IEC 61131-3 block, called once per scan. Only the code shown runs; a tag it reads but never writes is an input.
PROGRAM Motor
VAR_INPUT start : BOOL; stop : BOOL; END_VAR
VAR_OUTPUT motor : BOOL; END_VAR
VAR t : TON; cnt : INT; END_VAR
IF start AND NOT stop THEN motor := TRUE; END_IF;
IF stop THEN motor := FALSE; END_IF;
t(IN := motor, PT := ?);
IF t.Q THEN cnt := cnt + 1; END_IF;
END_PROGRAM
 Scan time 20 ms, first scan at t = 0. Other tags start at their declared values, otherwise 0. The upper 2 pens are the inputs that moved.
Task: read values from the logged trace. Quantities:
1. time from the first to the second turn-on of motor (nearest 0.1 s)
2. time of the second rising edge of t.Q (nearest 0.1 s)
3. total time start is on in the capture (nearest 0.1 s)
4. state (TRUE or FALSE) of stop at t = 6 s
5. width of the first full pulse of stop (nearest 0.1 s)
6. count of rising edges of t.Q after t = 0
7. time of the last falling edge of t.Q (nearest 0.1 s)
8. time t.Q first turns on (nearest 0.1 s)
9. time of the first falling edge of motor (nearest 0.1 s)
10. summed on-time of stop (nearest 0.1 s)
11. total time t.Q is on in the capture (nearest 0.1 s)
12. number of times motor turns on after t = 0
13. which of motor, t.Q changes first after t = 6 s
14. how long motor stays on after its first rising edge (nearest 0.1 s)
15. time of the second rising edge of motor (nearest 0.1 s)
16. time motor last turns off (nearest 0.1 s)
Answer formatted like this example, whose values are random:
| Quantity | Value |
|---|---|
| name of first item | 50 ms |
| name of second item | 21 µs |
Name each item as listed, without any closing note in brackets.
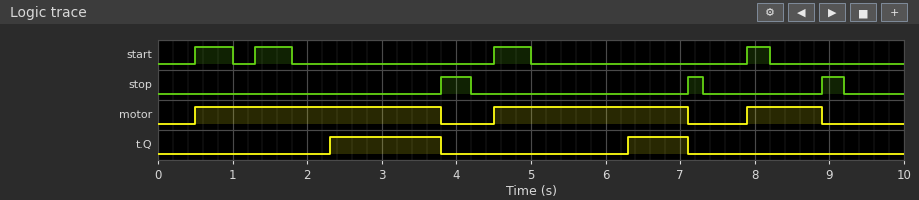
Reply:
| Quantity | Value |
|---|---|
| time from the first to the second turn-on of motor | 4.0 s |
| time of the second rising edge of t.Q | 6.3 s |
| total time start is on in the capture | 1.8 s |
| state (TRUE or FALSE) of stop at t = 6 s | FALSE |
| width of the first full pulse of stop | 0.4 s |
| count of rising edges of t.Q after t = 0 | 2 |
| time of the last falling edge of t.Q | 7.1 s |
| time t.Q first turns on | 2.3 s |
| time of the first falling edge of motor | 3.8 s |
| summed on-time of stop | 0.9 s |
| total time t.Q is on in the capture | 2.3 s |
| number of times motor turns on after t = 0 | 3 |
| which of motor, t.Q changes first after t = 6 s | t.Q |
| how long motor stays on after its first rising edge | 3.3 s |
| time of the second rising edge of motor | 4.5 s |
| time motor last turns off | 8.9 s |
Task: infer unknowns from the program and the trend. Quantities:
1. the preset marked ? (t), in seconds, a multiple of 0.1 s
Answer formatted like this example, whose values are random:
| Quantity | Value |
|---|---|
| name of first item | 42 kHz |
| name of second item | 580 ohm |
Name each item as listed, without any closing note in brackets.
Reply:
| Quantity | Value |
|---|---|
| the preset marked ? (t), in seconds, a multiple of 0.1 s | 1.8 s |
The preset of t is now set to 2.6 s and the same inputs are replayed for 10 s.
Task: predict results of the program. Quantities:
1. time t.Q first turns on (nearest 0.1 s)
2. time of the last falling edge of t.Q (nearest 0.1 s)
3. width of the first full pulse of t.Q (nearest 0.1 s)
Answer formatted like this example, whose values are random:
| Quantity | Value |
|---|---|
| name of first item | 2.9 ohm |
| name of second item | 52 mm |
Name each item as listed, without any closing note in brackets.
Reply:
| Quantity | Value |
|---|---|
| time t.Q first turns on | 3.1 s |
| time of the last falling edge of t.Q | 3.8 s |
| width of the first full pulse of t.Q | 0.7 s |
